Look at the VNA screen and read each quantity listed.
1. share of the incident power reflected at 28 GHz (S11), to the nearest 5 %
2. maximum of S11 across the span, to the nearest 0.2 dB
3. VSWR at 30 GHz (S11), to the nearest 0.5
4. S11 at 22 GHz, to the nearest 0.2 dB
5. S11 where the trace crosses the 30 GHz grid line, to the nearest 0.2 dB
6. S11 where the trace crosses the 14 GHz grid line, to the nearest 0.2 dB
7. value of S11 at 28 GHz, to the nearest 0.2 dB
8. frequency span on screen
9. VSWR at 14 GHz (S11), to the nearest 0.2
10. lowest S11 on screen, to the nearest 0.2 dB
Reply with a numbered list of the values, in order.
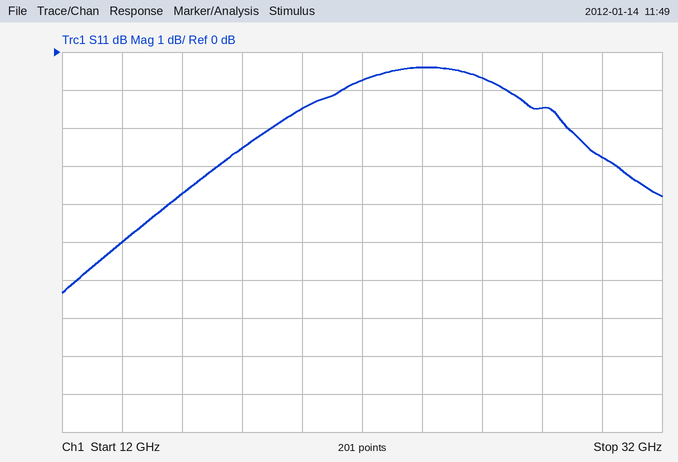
1. 70 %
2. -0.4 dB
3. 6.5
4. -0.8 dB
5. -2.8 dB
6. -5.0 dB
7. -1.4 dB
8. 20 GHz
9. 3.6
10. -6.4 dB
